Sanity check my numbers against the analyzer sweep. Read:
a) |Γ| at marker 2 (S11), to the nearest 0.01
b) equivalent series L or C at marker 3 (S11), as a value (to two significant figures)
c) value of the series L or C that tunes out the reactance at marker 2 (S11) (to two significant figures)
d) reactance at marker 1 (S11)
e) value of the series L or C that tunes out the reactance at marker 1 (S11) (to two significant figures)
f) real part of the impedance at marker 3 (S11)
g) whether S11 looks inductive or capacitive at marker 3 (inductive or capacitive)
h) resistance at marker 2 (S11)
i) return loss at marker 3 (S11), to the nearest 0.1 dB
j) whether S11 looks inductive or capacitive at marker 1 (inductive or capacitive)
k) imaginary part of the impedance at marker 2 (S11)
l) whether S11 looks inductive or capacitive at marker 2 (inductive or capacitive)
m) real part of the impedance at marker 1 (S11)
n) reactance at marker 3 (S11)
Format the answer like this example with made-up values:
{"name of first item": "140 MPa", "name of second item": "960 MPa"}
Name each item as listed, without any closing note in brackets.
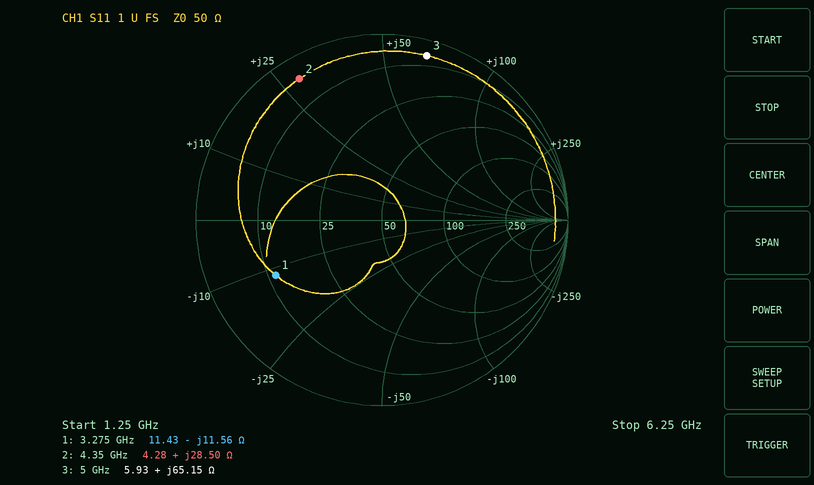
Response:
{"|Γ| at marker 2 (S11), to the nearest 0.01": "0.88", "equivalent series L or C at marker 3 (S11), as a value": "2.1 nH", "value of the series L or C that tunes out the reactance at marker 2 (S11)": "1.3 pF", "reactance at marker 1": "-11.56 Ω", "value of the series L or C that tunes out the reactance at marker 1 (S11)": "560 pH", "real part of the impedance at marker 3": "5.93 Ω", "whether S11 looks inductive or capacitive at marker 3": "inductive", "resistance at marker 2": "4.28 Ω", "return loss at marker 3 (S11), to the nearest 0.1 dB": "0.8 dB", "whether S11 looks inductive or capacitive at marker 1": "capacitive", "imaginary part of the impedance at marker 2": "+28.50 Ω", "whether S11 looks inductive or capacitive at marker 2": "inductive", "real part of the impedance at marker 1": "11.43 Ω", "reactance at marker 3": "+65.15 Ω"}
